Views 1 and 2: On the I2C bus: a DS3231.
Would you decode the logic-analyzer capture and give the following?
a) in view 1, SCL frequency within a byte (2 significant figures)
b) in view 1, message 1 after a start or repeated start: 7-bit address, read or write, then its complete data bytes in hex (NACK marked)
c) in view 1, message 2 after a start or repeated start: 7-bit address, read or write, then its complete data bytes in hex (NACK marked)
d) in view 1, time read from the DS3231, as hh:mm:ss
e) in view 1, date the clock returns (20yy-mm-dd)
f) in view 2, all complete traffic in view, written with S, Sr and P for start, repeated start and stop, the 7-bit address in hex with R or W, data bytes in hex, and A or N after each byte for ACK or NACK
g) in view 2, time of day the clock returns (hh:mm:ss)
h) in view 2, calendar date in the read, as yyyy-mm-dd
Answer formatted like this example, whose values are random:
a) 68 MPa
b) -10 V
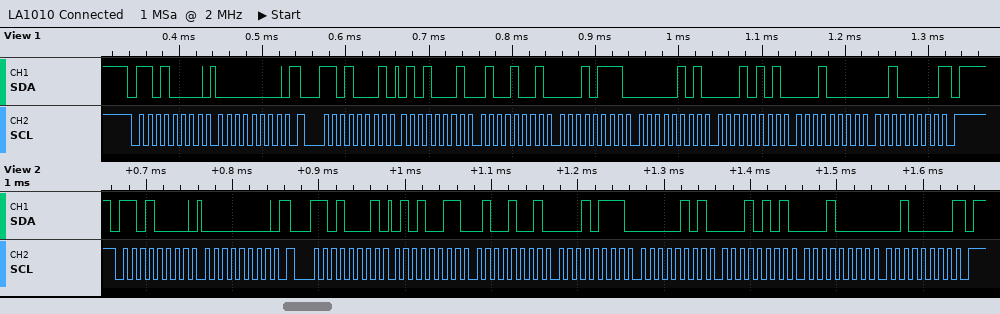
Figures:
a) 100 kHz
b) 0x68 write: 00
c) 0x68 read: 51 49 17 05 15 10 20 NACK
d) 17:49:51
e) 2020-10-15
f) S 68W A 00 A Sr 68R A 53 A 49 A 17 A 05 A 15 A 10 A 20 N P
g) 17:49:53
h) 2020-10-15
